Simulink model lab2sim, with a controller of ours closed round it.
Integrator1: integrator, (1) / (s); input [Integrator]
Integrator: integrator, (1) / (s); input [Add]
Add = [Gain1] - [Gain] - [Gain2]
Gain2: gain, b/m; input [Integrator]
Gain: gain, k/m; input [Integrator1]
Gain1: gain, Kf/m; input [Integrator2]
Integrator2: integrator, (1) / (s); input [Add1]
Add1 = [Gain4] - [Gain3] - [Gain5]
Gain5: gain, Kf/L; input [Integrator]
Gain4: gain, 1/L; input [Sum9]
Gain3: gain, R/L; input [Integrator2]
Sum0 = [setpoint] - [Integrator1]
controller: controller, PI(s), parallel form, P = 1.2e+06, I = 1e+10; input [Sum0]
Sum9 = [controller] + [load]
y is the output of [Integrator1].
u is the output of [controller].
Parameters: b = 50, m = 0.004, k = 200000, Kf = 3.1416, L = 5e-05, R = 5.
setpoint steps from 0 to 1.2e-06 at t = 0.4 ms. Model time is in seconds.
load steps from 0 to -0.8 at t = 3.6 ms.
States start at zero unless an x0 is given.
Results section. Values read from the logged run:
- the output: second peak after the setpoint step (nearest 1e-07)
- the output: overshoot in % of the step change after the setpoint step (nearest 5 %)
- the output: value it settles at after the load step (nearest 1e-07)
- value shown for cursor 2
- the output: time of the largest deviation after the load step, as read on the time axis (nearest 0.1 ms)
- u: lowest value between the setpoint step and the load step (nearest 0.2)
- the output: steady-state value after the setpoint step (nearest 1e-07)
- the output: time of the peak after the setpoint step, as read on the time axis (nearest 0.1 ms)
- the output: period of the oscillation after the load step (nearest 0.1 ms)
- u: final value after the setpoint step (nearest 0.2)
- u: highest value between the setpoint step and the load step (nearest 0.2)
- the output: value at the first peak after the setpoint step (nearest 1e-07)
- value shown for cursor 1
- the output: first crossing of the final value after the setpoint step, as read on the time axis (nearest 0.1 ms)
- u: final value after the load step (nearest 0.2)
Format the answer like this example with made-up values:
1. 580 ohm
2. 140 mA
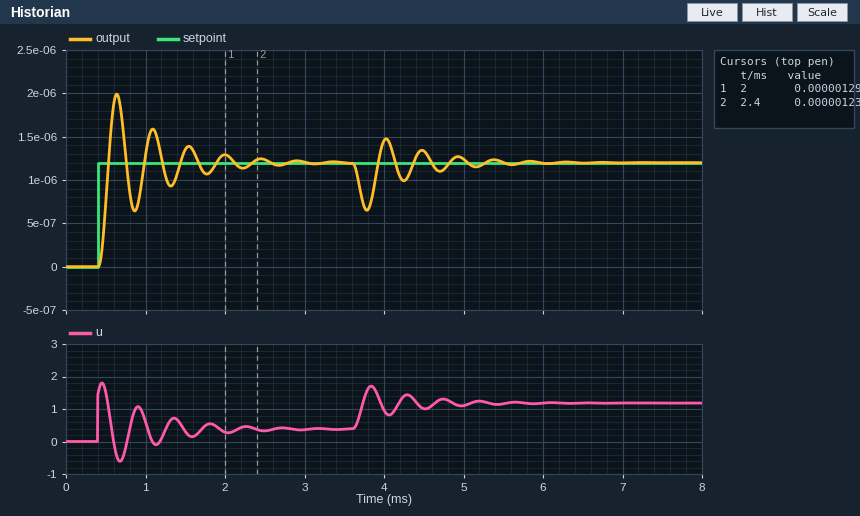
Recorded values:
1. 0.0000016
2. 65 %
3. 0.0000012
4. 0.000001235
5. 3.8 ms
6. -0.6
7. 0.0000012
8. 0.6 ms
9. 0.5 ms
10. 0.4
11. 1.8
12. 0.0000020
13. 0.000001290
14. 0.5 ms
15. 1.2
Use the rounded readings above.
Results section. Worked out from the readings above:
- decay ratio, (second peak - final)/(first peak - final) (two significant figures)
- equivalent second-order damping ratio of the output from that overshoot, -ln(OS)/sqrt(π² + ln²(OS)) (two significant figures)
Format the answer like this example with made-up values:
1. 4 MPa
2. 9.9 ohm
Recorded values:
1. 0.50
2. 0.14
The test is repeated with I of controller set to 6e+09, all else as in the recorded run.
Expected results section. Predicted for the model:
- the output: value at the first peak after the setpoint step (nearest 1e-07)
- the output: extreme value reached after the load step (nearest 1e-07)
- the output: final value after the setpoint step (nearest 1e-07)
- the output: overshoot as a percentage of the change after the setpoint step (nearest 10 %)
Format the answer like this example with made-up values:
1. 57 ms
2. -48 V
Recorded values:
1. 0.0000017
2. 0.0000006
3. 0.0000012
4. 40 %
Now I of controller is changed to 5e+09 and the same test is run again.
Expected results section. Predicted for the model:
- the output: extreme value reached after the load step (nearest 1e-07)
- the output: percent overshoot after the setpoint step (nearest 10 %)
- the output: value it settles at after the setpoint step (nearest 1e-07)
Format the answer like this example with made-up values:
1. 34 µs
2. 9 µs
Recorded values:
1. 0.0000006
2. 40 %
3. 0.0000012
